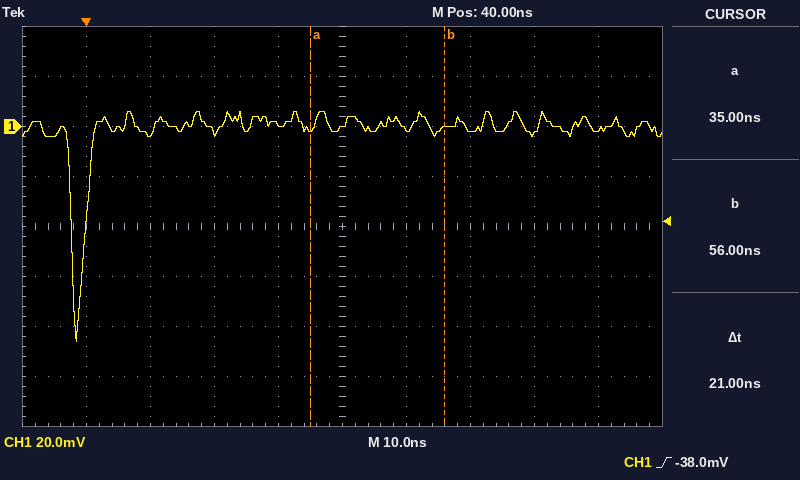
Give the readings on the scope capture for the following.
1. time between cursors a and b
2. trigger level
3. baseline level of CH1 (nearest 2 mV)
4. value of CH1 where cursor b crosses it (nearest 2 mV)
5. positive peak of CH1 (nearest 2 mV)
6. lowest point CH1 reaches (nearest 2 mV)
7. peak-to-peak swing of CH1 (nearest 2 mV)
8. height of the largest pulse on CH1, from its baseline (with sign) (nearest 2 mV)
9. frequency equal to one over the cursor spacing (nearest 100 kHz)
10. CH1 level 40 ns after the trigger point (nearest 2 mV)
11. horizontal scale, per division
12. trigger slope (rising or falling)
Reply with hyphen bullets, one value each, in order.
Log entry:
- 21 ns
- -38.0 mV
- 0 mV
- 0 mV
- 6 mV
- -86 mV
- 92 mV
- -86 mV
- 47.6 MHz
- 0 mV
- 10 ns
- rising
